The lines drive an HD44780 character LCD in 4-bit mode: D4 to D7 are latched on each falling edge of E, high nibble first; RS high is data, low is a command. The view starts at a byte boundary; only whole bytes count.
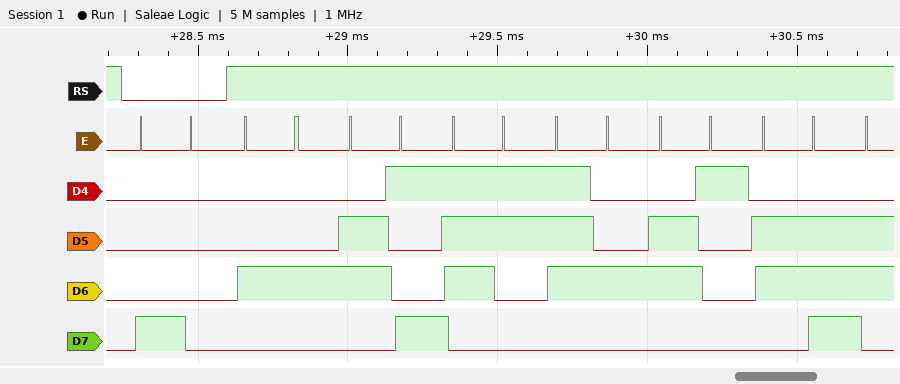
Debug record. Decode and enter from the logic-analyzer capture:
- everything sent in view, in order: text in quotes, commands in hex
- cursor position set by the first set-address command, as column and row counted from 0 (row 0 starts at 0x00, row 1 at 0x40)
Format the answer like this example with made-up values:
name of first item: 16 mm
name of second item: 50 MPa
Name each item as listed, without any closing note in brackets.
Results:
everything sent in view, in order: text in quotes, commands in hex: 0x80 "Distan"
cursor position set by the first set-address command, as column and row counted from 0: column 0, row 0
